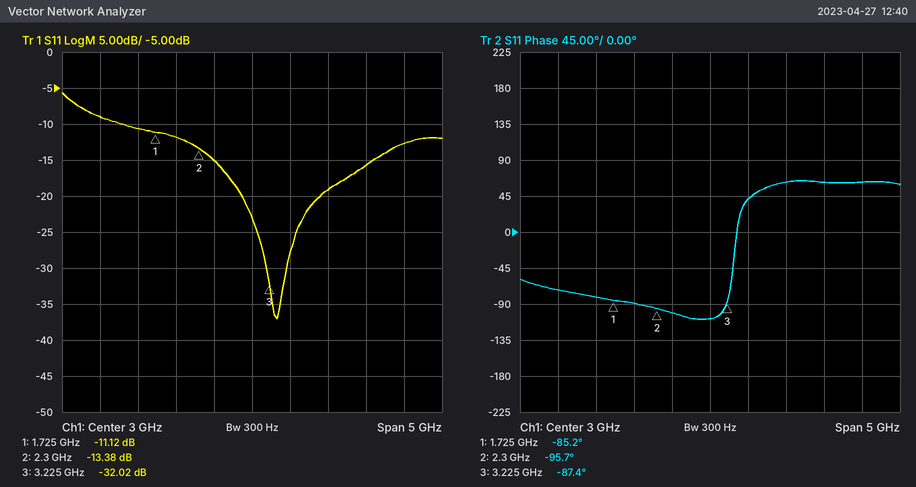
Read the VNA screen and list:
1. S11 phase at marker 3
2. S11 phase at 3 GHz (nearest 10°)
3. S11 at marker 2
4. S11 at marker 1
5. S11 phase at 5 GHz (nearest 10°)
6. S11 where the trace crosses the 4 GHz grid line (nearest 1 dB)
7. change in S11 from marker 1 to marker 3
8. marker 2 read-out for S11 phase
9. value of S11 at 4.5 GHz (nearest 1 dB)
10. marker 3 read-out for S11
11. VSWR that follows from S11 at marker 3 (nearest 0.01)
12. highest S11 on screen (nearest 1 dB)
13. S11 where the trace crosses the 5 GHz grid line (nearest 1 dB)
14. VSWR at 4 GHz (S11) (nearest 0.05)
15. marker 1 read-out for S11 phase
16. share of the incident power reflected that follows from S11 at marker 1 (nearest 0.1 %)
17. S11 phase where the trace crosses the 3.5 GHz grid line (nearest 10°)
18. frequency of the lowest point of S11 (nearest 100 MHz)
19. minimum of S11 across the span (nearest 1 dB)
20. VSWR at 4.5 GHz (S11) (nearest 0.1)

-87.4°
-110°
-13.38 dB
-11.12 dB
60°
-19 dB
-20.90 dB
-95.7°
-16 dB
-32.02 dB
1.05
-6 dB
-13 dB
1.25
-85.2°
7.7 %
40°
3.3 GHz
-37 dB
1.4
